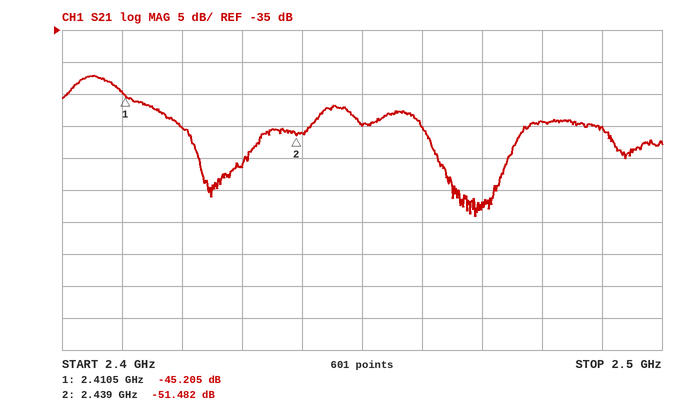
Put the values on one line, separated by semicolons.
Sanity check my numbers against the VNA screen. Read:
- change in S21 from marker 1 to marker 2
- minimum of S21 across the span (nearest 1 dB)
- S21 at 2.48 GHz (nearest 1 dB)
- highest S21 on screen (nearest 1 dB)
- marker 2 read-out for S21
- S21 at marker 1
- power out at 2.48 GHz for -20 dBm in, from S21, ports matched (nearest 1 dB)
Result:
-6.277 dB; -64 dB; -49 dB; -42 dB; -51.482 dB; -45.205 dB; -69 dBm
